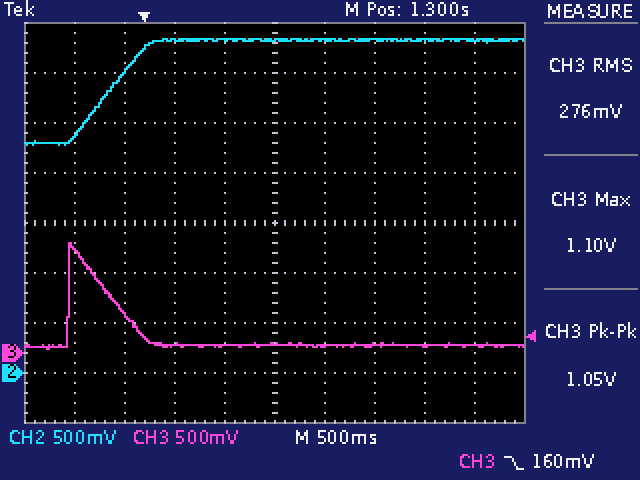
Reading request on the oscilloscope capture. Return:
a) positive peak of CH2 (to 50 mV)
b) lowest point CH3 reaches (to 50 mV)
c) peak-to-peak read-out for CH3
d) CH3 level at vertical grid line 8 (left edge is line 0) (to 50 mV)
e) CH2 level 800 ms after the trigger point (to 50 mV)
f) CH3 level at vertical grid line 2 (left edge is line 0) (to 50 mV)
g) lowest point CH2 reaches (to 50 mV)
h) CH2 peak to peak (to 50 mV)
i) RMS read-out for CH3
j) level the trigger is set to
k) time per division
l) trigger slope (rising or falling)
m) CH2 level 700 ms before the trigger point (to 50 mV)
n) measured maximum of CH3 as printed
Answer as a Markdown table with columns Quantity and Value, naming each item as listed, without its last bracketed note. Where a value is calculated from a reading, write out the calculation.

| Quantity | Value |
|---|---|
| positive peak of CH2 | 3.35 V |
| lowest point CH3 reaches | 50 mV |
| peak-to-peak read-out for CH3 | 1.05 V |
| CH3 level at vertical grid line 8 (left edge is line 0) | 50 mV |
| CH2 level 800 ms after the trigger point | 3.35 V |
| CH3 level at vertical grid line 2 (left edge is line 0) | 400 mV |
| lowest point CH2 reaches | 2.30 V |
| CH2 peak to peak | 3.35 V − (2.30 V) = 1.05 V |
| RMS read-out for CH3 | 276 mV |
| level the trigger is set to | 160 mV |
| time per division | 500 ms |
| trigger slope | falling |
| CH2 level 700 ms before the trigger point | 2.35 V |
| measured maximum of CH3 as printed | 1.10 V |
